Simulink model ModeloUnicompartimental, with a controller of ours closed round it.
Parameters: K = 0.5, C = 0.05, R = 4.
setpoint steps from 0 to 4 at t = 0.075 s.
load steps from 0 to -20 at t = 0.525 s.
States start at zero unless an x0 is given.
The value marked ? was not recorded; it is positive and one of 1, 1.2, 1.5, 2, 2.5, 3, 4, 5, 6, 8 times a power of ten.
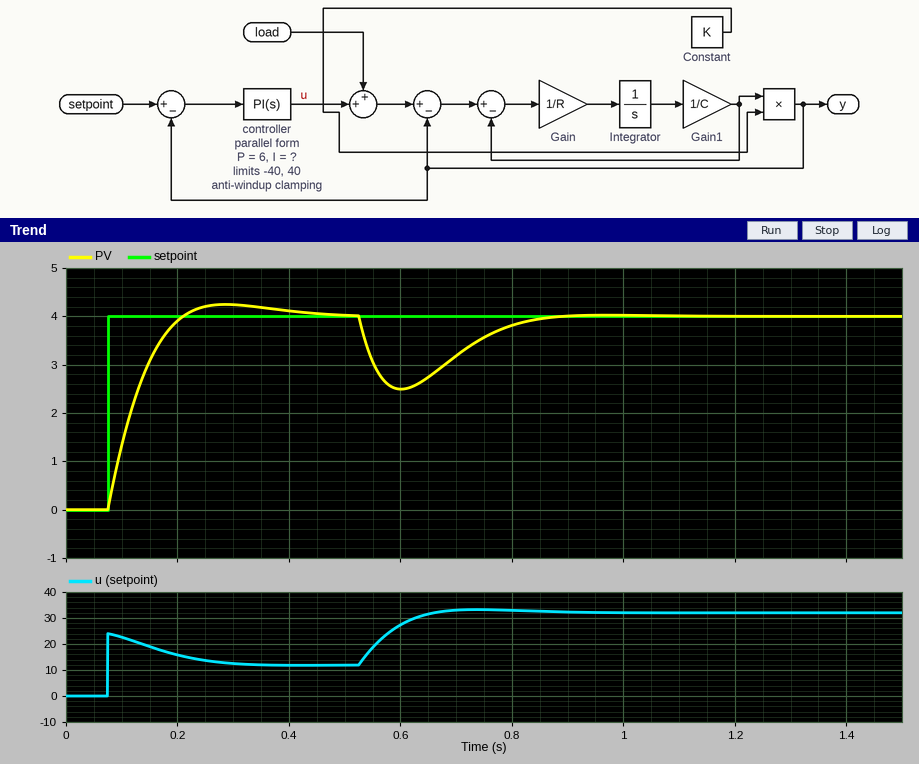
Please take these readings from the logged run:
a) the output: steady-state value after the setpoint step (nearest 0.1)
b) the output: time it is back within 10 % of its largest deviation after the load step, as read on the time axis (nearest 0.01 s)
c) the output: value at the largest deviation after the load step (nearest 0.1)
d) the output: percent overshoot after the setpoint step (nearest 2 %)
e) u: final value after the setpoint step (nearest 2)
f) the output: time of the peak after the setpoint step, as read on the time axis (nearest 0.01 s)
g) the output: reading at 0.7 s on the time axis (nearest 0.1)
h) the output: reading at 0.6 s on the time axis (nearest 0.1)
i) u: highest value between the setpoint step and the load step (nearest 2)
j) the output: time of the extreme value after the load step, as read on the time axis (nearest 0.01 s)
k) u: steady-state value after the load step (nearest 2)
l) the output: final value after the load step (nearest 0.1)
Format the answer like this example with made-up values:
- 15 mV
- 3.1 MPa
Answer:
- 4.0
- 0.81 s
- 2.5
- 6 %
- 12
- 0.29 s
- 3.2
- 2.5
- 24
- 0.60 s
- 32
- 4.0
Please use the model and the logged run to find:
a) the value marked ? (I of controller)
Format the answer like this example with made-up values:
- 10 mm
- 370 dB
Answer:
- 80
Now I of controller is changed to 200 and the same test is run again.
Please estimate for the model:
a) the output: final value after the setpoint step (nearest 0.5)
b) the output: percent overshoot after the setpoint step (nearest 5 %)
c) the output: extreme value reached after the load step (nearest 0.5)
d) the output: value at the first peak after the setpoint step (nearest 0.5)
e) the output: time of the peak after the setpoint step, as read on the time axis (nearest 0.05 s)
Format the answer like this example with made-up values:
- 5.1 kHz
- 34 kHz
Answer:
- 4.0
- 20 %
- 3.0
- 5.0
- 0.20 s
